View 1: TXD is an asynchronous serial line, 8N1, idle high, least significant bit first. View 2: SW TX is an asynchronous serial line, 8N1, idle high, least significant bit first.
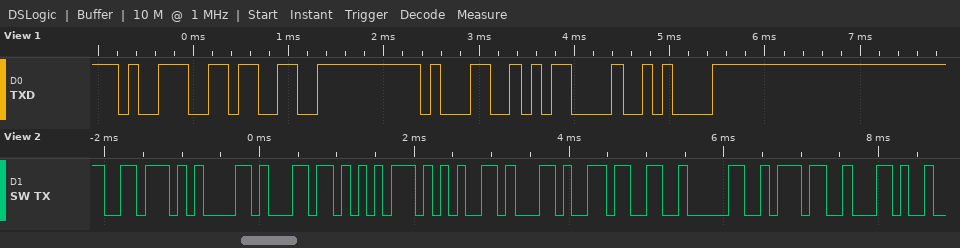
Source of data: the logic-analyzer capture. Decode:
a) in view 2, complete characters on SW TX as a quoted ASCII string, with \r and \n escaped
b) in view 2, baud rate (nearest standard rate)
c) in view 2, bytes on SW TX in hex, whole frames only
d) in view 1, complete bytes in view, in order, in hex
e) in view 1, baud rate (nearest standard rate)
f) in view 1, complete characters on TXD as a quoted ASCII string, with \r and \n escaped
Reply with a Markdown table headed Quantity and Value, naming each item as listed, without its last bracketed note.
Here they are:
| Quantity | Value |
|---|---|
| in view 2, complete characters on SW TX as a quoted ASCII string, with \r and \n escaped | "value,307," |
| in view 2, baud rate | 9600 baud |
| in view 2, bytes on SW TX in hex, whole frames only | 76 61 6C 75 65 2C 33 30 37 2C |
| in view 1, complete bytes in view, in order, in hex | 39 33 31 0D 0A |
| in view 1, baud rate | 9600 baud |
| in view 1, complete characters on TXD as a quoted ASCII string, with \r and \n escaped | "931\r\n" |
